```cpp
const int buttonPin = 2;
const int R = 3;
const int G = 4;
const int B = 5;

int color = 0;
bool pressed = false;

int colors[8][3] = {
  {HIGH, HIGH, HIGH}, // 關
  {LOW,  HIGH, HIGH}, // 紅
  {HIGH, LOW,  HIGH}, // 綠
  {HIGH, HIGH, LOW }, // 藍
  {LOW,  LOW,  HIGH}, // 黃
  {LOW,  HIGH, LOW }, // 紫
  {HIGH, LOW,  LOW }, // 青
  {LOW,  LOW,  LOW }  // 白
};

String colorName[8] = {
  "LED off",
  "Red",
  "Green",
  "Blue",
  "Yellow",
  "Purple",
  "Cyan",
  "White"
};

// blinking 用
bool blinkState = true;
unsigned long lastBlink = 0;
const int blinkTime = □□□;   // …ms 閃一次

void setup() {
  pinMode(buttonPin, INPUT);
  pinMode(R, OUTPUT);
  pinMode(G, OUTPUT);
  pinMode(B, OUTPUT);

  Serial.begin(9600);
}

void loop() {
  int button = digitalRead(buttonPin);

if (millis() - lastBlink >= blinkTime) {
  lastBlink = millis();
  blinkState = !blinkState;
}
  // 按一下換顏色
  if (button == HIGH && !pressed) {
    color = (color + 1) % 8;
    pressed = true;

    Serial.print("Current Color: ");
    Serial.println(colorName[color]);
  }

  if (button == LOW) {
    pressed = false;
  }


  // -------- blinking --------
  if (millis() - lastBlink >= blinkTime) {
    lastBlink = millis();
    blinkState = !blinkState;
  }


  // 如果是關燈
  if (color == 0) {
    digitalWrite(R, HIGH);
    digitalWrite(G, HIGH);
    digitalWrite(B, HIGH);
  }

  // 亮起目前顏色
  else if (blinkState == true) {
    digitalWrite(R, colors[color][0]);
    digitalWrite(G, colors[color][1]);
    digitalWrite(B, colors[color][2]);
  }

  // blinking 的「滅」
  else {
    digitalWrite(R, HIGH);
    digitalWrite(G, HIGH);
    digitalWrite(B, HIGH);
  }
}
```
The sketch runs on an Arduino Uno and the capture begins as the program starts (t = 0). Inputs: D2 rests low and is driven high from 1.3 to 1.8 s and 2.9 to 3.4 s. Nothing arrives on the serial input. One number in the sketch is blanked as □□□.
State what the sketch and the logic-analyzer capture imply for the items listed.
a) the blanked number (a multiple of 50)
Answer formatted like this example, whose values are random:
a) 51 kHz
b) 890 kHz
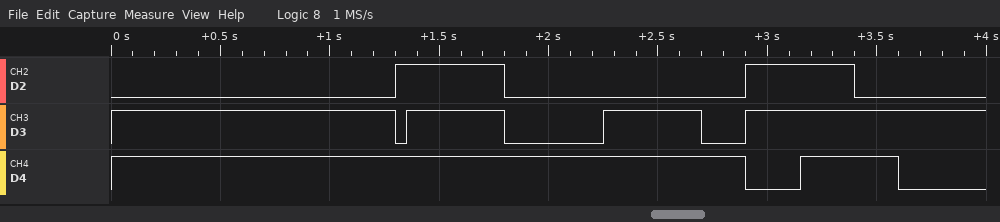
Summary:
a) 450
